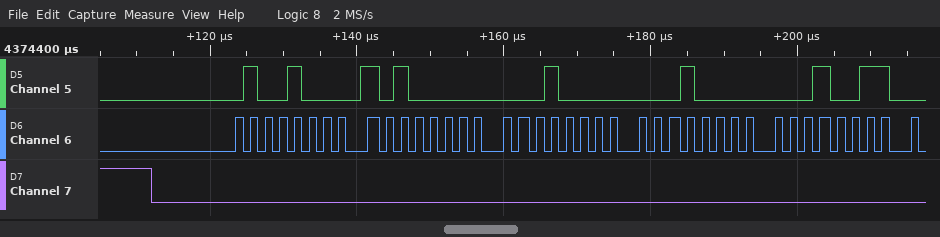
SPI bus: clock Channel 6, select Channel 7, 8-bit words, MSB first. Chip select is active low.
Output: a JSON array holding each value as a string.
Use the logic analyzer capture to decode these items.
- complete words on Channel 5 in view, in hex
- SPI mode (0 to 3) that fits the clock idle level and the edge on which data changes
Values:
["48, A0, 10, 10, 13", "0"]
